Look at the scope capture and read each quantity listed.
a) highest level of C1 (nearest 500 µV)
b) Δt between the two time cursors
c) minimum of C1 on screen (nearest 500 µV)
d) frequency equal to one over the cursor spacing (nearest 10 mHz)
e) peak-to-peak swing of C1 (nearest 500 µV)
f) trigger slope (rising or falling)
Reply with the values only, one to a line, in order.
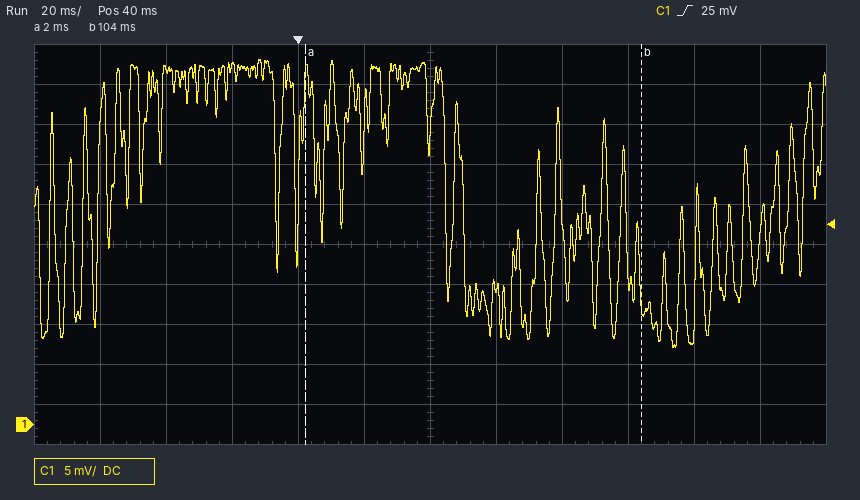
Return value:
45.5 mV
102 ms
9.5 mV
9.80 Hz
36.0 mV
rising
